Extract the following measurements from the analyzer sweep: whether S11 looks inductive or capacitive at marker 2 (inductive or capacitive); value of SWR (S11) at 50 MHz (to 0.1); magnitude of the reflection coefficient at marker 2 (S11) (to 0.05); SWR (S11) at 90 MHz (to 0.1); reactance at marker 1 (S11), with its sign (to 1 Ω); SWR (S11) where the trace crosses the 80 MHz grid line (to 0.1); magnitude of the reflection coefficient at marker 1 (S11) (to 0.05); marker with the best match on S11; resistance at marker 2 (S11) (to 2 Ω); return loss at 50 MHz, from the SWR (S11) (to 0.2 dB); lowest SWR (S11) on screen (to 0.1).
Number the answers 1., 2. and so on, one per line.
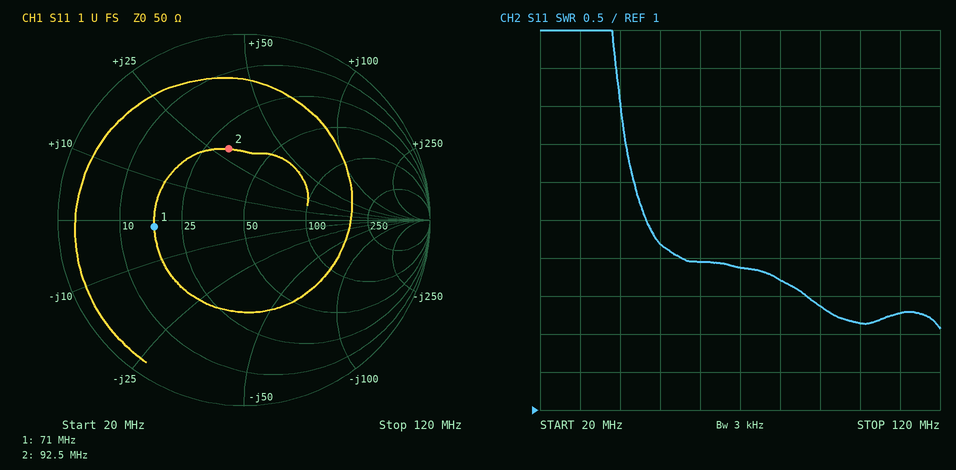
1. inductive
2. 3.2
3. 0.40
4. 2.4
5. -2 Ω
6. 2.7
7. 0.50
8. marker 2
9. 32 Ω
10. 5.6 dB
11. 2.1
